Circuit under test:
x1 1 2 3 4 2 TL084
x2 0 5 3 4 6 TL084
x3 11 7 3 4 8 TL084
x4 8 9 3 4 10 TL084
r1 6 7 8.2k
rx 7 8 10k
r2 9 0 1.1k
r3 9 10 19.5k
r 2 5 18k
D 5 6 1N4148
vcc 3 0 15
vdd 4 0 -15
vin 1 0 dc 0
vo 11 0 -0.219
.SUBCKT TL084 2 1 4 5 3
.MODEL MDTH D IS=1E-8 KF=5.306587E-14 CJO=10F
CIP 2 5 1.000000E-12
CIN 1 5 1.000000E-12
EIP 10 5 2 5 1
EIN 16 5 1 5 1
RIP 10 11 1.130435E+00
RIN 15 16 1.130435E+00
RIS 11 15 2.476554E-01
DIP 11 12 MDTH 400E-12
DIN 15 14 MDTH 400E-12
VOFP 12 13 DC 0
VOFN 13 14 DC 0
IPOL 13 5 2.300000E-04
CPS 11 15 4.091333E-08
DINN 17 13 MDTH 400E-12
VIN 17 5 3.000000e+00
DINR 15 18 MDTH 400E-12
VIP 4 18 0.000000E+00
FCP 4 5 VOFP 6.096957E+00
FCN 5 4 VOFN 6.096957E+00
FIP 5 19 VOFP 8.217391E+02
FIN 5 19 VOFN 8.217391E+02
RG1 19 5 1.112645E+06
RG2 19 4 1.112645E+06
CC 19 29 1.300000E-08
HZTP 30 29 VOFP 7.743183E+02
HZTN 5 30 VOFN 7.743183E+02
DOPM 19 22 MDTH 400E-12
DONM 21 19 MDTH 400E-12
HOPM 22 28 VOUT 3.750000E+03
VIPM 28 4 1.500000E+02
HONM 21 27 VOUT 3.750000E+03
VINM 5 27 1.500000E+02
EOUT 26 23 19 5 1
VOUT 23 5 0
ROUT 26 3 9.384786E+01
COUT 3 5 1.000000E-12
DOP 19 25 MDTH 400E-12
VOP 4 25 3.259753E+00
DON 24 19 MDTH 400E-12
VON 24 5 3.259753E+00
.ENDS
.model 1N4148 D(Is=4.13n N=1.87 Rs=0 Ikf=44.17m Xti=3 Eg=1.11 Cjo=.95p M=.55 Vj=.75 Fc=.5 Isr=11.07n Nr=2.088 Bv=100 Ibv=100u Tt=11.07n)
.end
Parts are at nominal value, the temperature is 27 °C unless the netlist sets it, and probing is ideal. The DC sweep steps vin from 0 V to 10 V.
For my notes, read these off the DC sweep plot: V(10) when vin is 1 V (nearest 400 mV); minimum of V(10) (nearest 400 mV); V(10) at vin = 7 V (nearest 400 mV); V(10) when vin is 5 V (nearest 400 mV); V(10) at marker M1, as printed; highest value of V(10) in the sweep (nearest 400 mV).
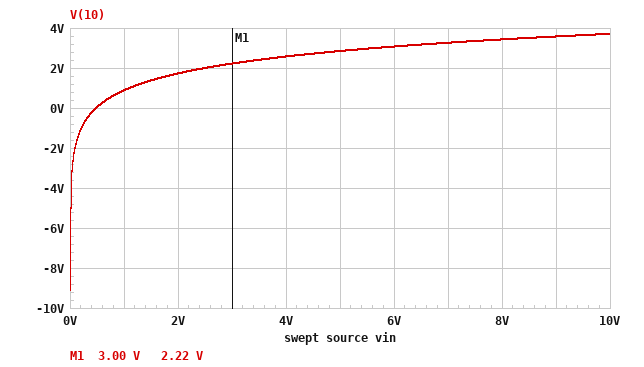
800 mV
-9.2 V
3.2 V
2.8 V
2.22 V
3.6 V
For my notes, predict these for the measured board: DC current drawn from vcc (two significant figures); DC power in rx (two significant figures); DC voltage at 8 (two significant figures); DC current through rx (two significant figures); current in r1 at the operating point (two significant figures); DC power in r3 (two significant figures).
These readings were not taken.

5.7 mA
7.1 µW
-490 mV
27 µA
27 µA
3.8 mW
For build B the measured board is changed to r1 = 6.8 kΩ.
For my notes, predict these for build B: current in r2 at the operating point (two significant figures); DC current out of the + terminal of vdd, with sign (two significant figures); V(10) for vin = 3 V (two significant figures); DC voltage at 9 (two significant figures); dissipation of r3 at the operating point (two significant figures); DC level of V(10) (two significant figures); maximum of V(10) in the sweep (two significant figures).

490 µA
-6.2 mA
3.5 V
-540 mV
4.7 mW
-10 V
5.3 V
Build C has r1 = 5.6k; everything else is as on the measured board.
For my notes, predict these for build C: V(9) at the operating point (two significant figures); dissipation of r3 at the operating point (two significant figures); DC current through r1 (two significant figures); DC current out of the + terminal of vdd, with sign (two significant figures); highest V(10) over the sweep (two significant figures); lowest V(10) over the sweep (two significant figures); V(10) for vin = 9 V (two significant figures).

-610 mV
6.0 mW
39 µA
-6.2 mA
7.3 V
-11 V
7.1 V
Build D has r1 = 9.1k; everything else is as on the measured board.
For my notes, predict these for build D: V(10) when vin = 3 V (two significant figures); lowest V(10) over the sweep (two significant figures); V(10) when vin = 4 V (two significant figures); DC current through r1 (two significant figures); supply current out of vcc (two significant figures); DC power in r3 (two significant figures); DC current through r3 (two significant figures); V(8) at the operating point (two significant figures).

1.6 V
-8.6 V
1.9 V
24 µA
5.7 mA
3.4 mW
420 µA
-460 mV
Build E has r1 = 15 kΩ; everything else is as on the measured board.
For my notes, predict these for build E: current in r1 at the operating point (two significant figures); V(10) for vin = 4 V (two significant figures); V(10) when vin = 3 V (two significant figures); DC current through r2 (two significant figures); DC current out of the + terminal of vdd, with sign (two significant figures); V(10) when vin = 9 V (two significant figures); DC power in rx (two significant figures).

15 µA
-450 mV
-640 mV
330 µA
-6.0 mA
96 mV
2.1 µW
